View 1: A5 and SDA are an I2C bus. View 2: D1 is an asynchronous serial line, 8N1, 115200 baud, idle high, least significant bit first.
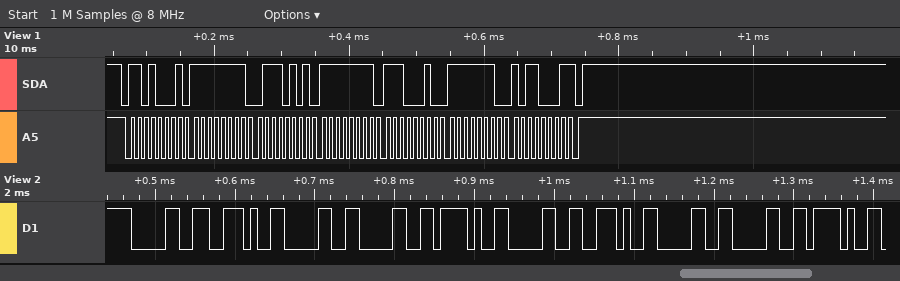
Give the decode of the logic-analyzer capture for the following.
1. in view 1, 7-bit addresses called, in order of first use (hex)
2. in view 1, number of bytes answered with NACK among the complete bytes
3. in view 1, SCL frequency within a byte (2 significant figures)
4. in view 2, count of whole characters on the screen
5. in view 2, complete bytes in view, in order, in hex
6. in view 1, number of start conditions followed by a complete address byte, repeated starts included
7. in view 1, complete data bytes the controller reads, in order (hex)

0x68
1
100 kHz
10
30 2E 30 30 2F 30 2E 30 30 2F
1
FF 75 FF E2 FE B1
